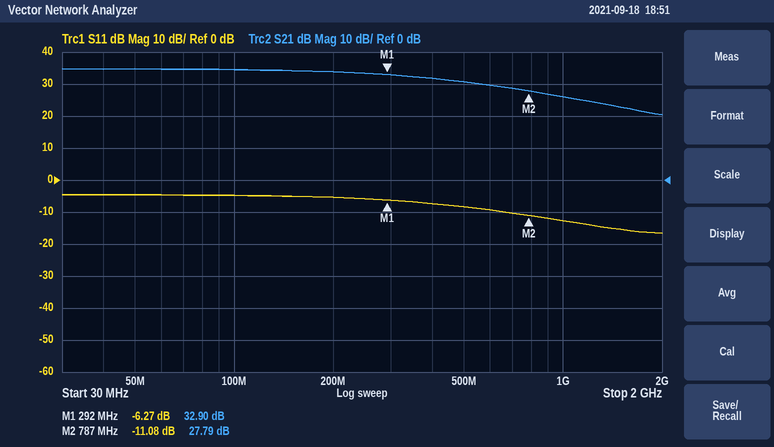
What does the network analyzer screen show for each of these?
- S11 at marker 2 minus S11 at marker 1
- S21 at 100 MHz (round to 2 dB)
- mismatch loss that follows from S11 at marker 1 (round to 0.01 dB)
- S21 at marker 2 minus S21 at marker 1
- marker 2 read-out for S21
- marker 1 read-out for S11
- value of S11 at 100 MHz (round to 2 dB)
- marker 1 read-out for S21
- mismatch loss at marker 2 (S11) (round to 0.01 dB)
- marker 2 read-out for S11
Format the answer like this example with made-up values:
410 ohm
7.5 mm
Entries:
-4.81 dB
34 dB
1.17 dB
-5.11 dB
27.79 dB
-6.27 dB
-4 dB
32.90 dB
0.35 dB
-11.08 dB
